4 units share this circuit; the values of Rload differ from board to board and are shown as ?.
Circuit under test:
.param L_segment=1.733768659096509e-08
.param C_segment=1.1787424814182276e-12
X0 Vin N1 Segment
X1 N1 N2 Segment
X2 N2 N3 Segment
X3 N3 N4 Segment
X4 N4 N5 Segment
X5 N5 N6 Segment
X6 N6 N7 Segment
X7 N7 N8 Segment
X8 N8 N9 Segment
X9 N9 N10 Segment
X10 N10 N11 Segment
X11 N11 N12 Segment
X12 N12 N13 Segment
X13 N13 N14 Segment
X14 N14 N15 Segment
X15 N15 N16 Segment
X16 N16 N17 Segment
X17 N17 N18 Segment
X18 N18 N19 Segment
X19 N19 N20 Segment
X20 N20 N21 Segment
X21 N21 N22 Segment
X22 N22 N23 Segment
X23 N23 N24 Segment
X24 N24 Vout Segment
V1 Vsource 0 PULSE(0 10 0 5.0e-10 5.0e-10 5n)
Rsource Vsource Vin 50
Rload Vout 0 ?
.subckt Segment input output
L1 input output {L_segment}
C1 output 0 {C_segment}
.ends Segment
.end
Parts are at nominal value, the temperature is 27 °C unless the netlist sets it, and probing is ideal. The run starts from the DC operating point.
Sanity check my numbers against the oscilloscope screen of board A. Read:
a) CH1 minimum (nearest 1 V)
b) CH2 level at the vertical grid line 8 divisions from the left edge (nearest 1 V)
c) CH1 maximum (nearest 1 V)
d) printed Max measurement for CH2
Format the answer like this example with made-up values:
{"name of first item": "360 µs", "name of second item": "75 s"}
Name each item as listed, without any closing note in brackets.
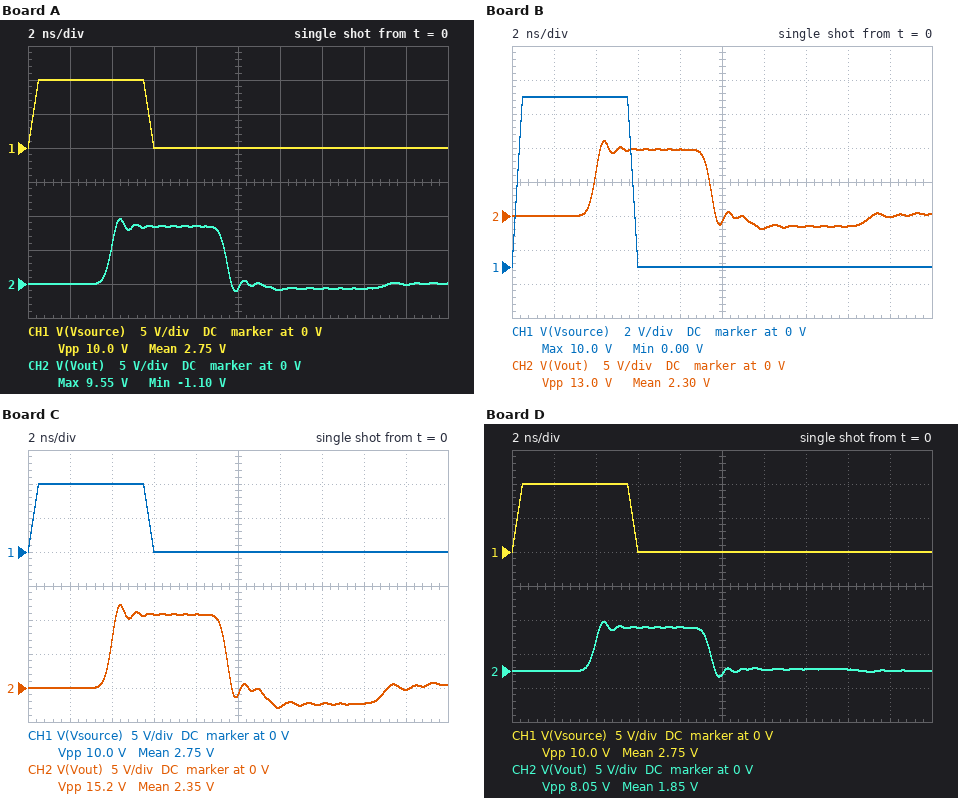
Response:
{"CH1 minimum": "0 V", "CH2 level at the vertical grid line 8 divisions from the left edge": "-1 V", "CH1 maximum": "10 V", "printed Max measurement for CH2": "9.55 V"}
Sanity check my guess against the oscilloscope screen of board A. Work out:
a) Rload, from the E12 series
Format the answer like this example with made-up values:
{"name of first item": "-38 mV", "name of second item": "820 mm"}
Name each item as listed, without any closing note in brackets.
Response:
{"Rload, from the E12 series": "180 Ω"}
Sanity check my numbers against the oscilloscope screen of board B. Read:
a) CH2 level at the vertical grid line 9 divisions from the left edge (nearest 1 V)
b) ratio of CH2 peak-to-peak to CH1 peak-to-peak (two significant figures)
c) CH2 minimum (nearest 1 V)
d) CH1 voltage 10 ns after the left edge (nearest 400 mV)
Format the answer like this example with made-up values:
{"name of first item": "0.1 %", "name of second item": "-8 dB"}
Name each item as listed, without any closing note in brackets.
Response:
{"CH2 level at the vertical grid line 9 divisions from the left edge": "0 V", "ratio of CH2 peak-to-peak to CH1 peak-to-peak": "1.3", "CH2 minimum": "-2 V", "CH1 voltage 10 ns after the left edge": "0 V"}
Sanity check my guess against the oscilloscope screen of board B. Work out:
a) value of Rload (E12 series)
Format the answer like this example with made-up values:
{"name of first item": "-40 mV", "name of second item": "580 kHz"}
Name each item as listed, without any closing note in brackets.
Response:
{"value of Rload": "270 Ω"}
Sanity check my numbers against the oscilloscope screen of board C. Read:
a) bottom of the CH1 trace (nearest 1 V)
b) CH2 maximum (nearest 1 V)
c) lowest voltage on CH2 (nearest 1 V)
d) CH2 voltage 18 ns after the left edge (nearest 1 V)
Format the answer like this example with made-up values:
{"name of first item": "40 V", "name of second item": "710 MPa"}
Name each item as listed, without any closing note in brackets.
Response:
{"bottom of the CH1 trace": "0 V", "CH2 maximum": "12 V", "lowest voltage on CH2": "-3 V", "CH2 voltage 18 ns after the left edge": "0 V"}
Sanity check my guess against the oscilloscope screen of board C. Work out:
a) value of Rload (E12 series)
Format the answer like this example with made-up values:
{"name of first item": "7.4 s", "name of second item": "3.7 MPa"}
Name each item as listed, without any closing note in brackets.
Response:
{"value of Rload": "390 Ω"}
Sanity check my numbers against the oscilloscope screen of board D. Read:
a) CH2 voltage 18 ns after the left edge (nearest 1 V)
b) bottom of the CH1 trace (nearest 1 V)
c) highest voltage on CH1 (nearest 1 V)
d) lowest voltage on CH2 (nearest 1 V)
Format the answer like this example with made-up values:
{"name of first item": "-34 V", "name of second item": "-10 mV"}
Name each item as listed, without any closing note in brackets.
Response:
{"CH2 voltage 18 ns after the left edge": "0 V", "bottom of the CH1 trace": "0 V", "highest voltage on CH1": "10 V", "lowest voltage on CH2": "-1 V"}
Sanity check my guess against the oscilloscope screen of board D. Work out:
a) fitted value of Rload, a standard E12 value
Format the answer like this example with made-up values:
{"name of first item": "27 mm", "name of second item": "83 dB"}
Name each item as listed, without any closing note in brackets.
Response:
{"fitted value of Rload, a standard E12 value": "100 Ω"}
